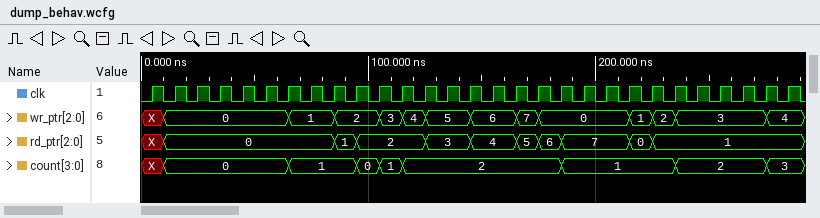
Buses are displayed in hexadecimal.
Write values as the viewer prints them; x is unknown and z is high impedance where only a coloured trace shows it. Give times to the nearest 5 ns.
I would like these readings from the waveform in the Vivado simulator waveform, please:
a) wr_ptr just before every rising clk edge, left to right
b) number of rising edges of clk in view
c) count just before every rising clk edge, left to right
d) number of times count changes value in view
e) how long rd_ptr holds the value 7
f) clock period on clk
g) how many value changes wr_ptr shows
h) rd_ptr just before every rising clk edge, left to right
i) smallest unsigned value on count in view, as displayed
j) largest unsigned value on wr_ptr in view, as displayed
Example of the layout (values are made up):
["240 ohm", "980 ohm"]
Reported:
["X, 0, 0, 0, 0, 0, 0, 1, 1, 2, 2, 3, 4, 5, 5, 6, 6, 7, 0, 0, 0, 0, 1, 2, 3, 3, 3, 3, 4", "29", "X, 0, 0, 0, 0, 0, 0, 1, 1, 1, 0, 1, 2, 2, 2, 2, 2, 2, 2, 1, 1, 1, 1, 1, 2, 2, 2, 2, 3", "8", "30 ns", "10 ns", "13", "X, 0, 0, 0, 0, 0, 0, 0, 0, 1, 2, 2, 2, 3, 3, 4, 4, 5, 6, 7, 7, 7, 0, 1, 1, 1, 1, 1, 1", "0", "7"]
